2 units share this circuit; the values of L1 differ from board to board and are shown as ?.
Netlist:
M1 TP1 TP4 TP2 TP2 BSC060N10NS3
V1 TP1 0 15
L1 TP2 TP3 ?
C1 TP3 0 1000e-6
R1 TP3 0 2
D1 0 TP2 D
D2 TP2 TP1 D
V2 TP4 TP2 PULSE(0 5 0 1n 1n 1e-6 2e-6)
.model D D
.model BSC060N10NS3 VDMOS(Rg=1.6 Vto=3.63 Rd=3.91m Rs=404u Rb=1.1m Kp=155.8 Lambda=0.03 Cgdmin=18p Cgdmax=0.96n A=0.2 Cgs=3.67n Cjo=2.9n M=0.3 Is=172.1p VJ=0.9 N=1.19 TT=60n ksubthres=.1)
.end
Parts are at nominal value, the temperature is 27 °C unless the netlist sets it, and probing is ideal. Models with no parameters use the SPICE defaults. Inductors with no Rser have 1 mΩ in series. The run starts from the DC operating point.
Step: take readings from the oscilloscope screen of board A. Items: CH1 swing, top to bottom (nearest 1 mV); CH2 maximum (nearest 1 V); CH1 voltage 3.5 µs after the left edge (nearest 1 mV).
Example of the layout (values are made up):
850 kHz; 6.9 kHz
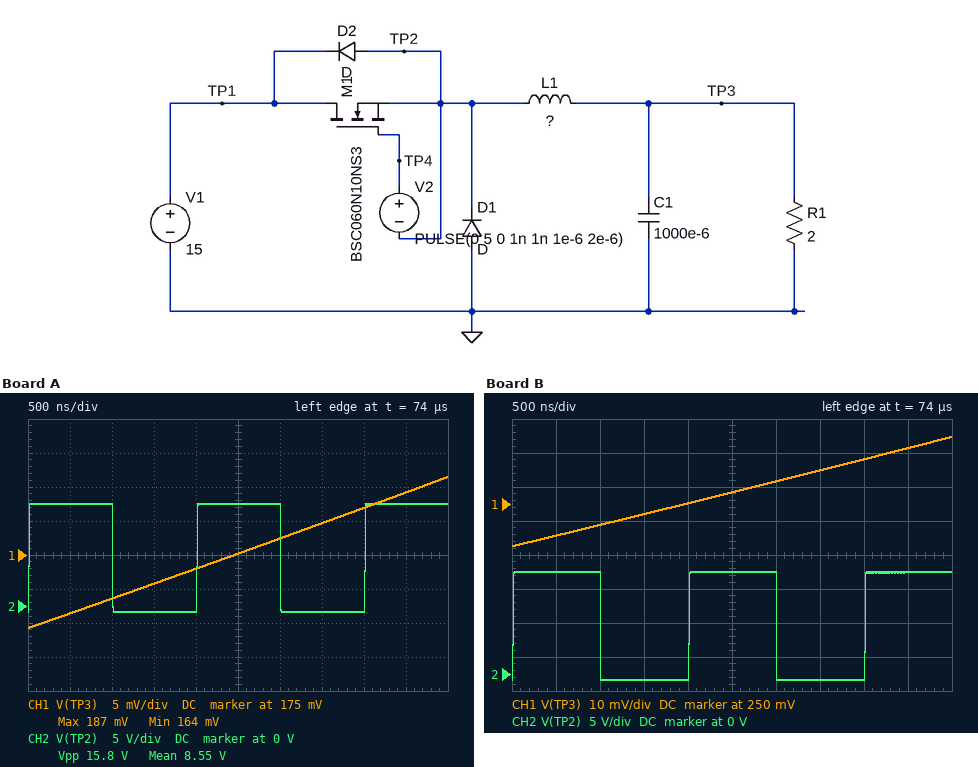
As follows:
22 mV; 15 V; 180 mV
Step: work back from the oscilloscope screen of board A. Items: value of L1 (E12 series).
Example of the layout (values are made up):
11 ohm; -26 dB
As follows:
120 µH
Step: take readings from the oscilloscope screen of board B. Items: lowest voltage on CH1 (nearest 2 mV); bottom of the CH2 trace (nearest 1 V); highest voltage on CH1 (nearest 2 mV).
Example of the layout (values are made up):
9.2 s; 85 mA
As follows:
238 mV; -1 V; 270 mV
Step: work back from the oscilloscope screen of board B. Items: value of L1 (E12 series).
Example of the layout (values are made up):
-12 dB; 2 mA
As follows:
82 µH
